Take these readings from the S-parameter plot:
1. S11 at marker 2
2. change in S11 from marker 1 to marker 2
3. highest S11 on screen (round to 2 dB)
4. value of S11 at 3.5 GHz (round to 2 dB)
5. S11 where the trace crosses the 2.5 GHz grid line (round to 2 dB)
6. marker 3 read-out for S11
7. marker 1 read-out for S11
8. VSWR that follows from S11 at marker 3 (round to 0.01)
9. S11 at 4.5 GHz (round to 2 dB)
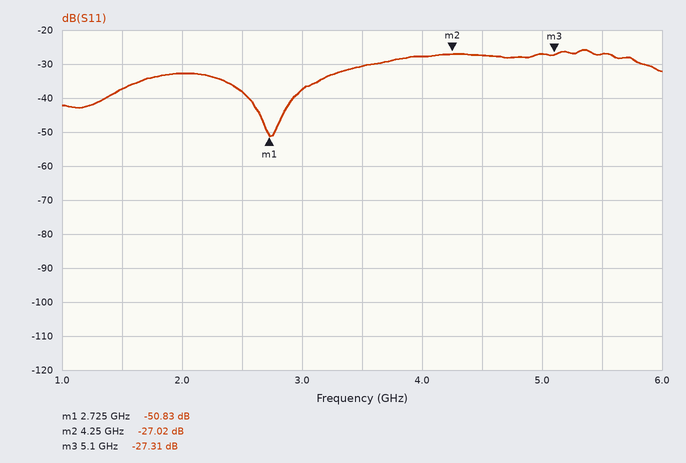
-27.02 dB
23.81 dB
-26 dB
-30 dB
-38 dB
-27.31 dB
-50.83 dB
1.09
-28 dB
